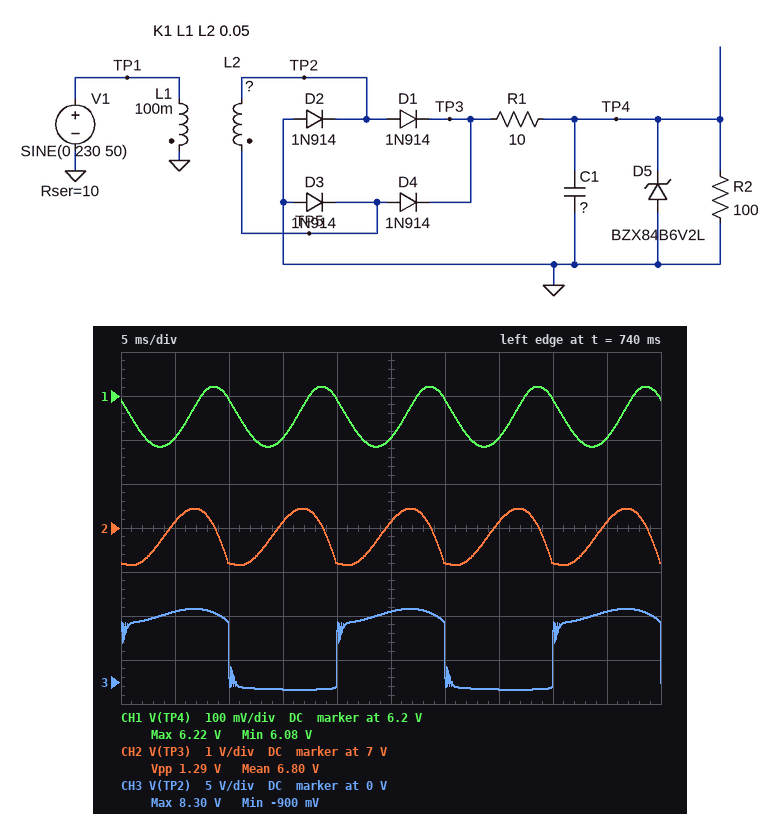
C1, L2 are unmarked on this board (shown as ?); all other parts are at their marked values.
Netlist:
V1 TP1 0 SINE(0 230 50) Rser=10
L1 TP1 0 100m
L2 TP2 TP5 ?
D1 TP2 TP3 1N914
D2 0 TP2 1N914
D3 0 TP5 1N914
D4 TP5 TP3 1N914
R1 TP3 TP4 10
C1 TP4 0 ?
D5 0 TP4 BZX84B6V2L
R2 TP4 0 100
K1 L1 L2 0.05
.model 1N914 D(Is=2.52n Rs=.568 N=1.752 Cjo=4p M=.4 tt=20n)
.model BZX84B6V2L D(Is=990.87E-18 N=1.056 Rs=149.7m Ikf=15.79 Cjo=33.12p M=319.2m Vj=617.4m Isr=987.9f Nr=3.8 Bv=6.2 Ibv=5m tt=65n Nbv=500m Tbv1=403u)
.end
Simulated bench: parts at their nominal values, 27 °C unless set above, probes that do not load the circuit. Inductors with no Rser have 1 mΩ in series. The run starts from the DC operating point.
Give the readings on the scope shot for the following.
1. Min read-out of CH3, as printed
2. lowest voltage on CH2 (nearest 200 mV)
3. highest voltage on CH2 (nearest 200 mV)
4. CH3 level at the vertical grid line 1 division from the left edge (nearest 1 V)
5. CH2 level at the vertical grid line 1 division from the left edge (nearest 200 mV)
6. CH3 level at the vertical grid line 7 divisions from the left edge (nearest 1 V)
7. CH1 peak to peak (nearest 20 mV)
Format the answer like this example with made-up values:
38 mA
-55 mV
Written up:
-900 mV
6.2 V
7.4 V
8 V
7.2 V
-1 V
140 mV
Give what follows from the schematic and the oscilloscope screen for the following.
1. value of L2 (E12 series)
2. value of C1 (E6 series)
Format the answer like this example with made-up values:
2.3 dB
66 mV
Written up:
150 mH
1.5 mF
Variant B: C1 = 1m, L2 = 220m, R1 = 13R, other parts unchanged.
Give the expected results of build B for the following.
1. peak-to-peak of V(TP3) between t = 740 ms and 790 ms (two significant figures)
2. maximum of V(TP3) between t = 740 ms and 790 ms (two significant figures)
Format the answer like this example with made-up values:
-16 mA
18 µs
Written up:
1.9 V
8.1 V
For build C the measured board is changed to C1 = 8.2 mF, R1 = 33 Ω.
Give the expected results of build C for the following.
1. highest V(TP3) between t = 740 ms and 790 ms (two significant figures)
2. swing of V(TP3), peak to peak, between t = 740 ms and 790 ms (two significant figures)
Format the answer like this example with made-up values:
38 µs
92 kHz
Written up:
8.7 V
3.9 V
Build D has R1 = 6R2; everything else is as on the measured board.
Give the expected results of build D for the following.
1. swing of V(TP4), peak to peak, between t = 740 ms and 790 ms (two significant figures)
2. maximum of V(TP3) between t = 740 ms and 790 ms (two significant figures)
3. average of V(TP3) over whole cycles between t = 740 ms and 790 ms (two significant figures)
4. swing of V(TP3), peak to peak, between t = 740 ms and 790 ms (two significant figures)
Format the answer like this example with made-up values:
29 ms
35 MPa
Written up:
140 mV
7.0 V
6.6 V
880 mV
